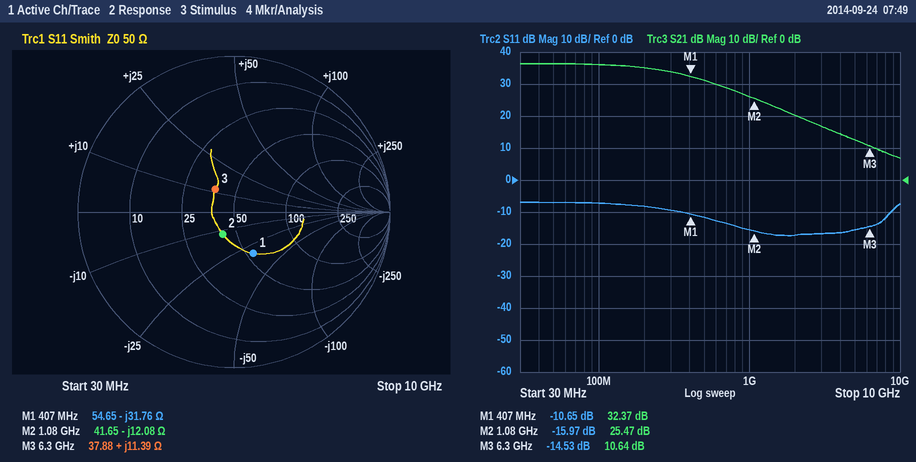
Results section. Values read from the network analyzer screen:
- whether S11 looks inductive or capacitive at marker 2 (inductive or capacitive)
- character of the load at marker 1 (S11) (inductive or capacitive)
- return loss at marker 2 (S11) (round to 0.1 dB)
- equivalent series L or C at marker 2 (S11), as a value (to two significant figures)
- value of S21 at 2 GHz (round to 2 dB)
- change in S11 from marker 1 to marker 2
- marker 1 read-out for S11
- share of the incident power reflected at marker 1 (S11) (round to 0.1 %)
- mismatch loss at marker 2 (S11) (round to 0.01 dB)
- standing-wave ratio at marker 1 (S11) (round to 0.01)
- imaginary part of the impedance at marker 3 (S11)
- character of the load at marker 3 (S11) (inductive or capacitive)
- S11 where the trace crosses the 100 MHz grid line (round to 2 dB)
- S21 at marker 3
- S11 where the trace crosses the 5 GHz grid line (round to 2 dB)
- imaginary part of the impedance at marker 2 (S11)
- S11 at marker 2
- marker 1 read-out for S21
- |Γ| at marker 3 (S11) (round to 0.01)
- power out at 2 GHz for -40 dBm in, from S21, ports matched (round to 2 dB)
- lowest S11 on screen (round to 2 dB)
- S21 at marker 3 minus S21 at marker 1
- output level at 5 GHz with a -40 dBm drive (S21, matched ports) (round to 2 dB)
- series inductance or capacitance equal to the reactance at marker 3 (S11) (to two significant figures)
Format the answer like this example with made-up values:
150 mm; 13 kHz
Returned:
capacitive; capacitive; 16.0 dB; 12 pF; 20 dB; -5.32 dB; -10.65 dB; 8.6 %; 0.11 dB; 1.83; +11.39 Ω; inductive; -8 dB; 10.64 dB; -16 dB; -12.08 Ω; -15.97 dB; 32.37 dB; 0.19; -20 dBm; -18 dB; -21.73 dB; -28 dBm; 290 pH
